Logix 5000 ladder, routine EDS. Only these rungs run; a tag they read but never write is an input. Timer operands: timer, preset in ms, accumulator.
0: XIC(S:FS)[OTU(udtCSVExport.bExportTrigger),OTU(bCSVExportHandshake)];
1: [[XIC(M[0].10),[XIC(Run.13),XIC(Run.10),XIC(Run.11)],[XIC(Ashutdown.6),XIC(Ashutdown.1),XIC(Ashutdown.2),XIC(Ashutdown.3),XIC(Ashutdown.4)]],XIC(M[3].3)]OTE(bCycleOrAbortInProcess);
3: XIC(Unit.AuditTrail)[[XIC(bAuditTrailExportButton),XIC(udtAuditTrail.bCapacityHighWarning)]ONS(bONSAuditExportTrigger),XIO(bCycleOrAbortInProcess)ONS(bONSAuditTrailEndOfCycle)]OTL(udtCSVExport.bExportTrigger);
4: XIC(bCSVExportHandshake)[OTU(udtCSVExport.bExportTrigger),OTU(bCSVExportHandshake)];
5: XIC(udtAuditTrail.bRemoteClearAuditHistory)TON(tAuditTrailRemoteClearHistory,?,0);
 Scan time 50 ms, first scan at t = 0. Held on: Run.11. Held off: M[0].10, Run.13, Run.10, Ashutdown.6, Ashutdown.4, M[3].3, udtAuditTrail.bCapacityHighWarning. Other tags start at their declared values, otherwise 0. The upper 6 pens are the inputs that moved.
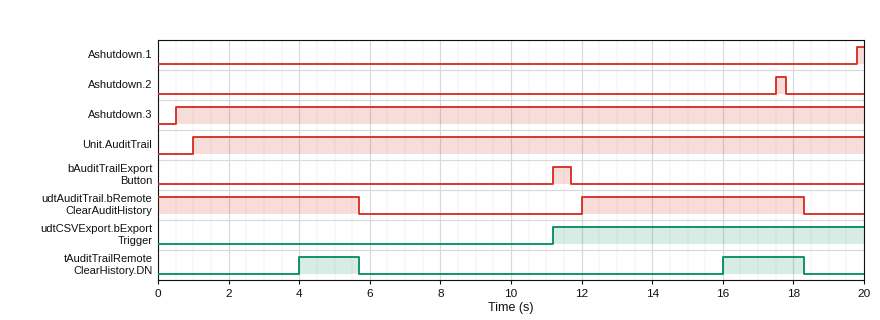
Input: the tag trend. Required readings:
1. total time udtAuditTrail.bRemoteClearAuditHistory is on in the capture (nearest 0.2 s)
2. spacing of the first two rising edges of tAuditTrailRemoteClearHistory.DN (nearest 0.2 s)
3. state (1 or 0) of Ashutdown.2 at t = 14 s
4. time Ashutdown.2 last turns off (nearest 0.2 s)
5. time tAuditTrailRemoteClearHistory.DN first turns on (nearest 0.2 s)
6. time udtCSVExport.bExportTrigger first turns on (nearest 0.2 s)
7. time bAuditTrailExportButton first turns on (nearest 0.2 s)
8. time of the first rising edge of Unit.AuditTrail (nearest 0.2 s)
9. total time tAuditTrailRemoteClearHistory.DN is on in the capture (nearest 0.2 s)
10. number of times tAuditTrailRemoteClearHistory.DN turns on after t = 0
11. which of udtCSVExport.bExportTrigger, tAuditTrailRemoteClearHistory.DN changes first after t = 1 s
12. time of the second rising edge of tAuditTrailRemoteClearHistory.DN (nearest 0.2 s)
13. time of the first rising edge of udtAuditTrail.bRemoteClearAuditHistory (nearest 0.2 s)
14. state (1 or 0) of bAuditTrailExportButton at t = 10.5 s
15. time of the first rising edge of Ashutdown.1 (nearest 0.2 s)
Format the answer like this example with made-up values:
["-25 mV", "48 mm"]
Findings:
["12.0 s", "12.0 s", "0", "17.8 s", "4.0 s", "11.2 s", "11.2 s", "1.0 s", "4.0 s", "2", "tAuditTrailRemoteClearHistory.DN", "16.0 s", "12.0 s", "0", "19.8 s"]
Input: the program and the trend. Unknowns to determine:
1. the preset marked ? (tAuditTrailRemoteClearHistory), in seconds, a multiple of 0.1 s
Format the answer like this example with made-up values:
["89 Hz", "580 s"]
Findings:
["4.0 s"]
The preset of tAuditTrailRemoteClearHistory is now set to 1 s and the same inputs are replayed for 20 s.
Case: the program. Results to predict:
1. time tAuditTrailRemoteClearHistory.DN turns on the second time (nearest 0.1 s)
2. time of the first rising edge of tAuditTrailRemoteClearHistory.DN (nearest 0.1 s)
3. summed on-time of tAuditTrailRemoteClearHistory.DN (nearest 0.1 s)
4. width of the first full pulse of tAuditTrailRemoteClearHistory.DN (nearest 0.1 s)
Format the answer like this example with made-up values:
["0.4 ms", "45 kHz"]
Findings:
["13.0 s", "1.0 s", "10.0 s", "4.7 s"]
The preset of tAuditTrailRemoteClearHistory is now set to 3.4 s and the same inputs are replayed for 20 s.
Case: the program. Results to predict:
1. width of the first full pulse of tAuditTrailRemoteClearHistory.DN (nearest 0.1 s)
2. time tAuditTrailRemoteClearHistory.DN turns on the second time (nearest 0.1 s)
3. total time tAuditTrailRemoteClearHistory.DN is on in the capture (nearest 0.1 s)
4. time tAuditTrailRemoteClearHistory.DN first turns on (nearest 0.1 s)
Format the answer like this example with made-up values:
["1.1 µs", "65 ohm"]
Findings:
["2.3 s", "15.4 s", "5.2 s", "3.4 s"]
